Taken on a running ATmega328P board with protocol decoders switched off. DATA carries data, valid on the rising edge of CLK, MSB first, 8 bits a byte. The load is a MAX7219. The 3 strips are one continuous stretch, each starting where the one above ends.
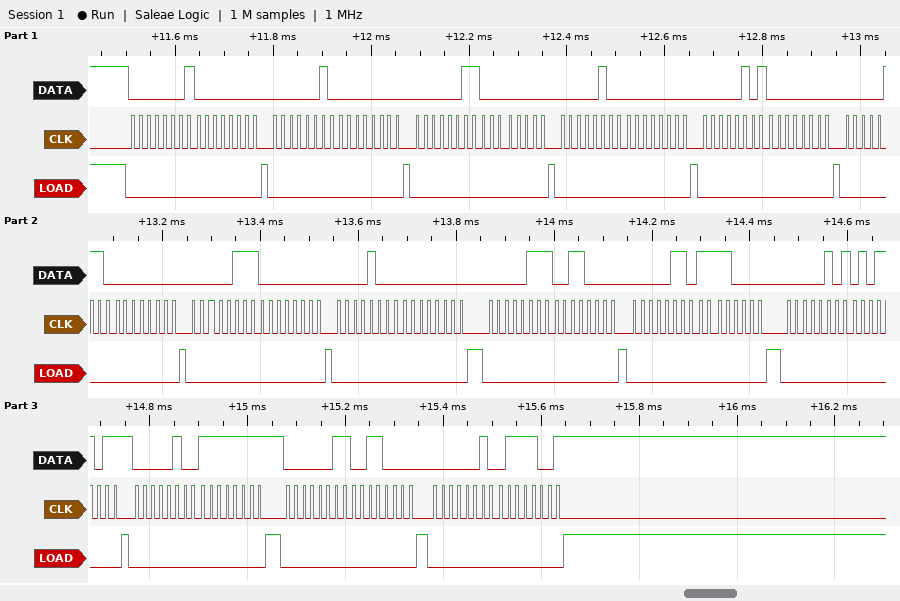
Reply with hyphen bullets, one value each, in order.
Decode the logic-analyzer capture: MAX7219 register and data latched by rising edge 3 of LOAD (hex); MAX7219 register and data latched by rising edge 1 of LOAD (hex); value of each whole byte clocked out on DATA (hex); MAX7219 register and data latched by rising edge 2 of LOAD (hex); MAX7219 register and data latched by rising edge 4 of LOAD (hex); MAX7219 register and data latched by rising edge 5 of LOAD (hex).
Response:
- register 0x3, data 0x00
- register 0x1, data 0x00
- 01 00 02 00 03 00 04 00 05 00 06 00 07 00 08 00 07 30 06 F0 05 5B 04 FF 03 30 02 79
- register 0x2, data 0x00
- register 0x4, data 0x00
- register 0x5, data 0x00
